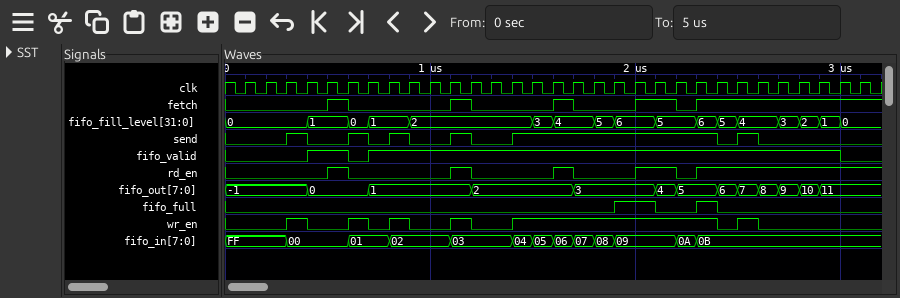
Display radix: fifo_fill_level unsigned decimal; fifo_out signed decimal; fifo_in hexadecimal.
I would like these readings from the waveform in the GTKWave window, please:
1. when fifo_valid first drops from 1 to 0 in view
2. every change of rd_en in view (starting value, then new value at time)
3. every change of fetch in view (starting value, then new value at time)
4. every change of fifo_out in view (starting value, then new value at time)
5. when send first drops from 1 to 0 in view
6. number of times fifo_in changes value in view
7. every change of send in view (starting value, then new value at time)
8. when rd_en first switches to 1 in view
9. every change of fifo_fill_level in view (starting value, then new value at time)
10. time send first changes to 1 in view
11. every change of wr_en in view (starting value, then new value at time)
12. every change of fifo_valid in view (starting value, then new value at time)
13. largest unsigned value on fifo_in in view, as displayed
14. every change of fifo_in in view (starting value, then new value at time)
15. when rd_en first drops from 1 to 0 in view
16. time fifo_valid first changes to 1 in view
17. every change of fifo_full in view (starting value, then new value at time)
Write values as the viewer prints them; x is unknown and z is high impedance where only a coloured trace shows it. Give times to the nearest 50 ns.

600 ns
0, 1 at 500 ns, 0 at 600 ns, 1 at 1100 ns, 0 at 1200 ns, 1 at 1600 ns, 0 at 1700 ns, 1 at 2000 ns, 0 at 2200 ns, 1 at 2300 ns
0, 1 at 500 ns, 0 at 600 ns, 1 at 1100 ns, 0 at 1200 ns, 1 at 1600 ns, 0 at 1700 ns, 1 at 2000 ns, 0 at 2200 ns, 1 at 2300 ns
-1, 0 at 400 ns, 1 at 700 ns, 2 at 1200 ns, 3 at 1700 ns, 4 at 2100 ns, 5 at 2200 ns, 6 at 2400 ns, 7 at 2500 ns, 8 at 2600 ns, 9 at 2700 ns, 10 at 2800 ns, 11 at 2900 ns
400 ns
12
0, 1 at 300 ns, 0 at 400 ns, 1 at 600 ns, 0 at 700 ns, 1 at 800 ns, 0 at 900 ns, 1 at 1100 ns, 0 at 1200 ns, 1 at 1400 ns, 0 at 2400 ns, 1 at 2500 ns, 0 at 2600 ns
500 ns
0, 1 at 400 ns, 0 at 600 ns, 1 at 700 ns, 2 at 900 ns, 3 at 1500 ns, 4 at 1600 ns, 5 at 1800 ns, 6 at 1900 ns, 5 at 2100 ns, 6 at 2300 ns, 5 at 2400 ns, 4 at 2500 ns, 3 at 2700 ns, 2 at 2800 ns, 1 at 2900 ns, 0 at 3000 ns
300 ns
0, 1 at 300 ns, 0 at 400 ns, 1 at 600 ns, 0 at 700 ns, 1 at 800 ns, 0 at 900 ns, 1 at 1100 ns, 0 at 1200 ns, 1 at 1400 ns, 0 at 2400 ns, 1 at 2500 ns, 0 at 2600 ns
0, 1 at 400 ns, 0 at 600 ns, 1 at 700 ns, 0 at 3000 ns
FF
FF, 00 at 300 ns, 01 at 600 ns, 02 at 800 ns, 03 at 1100 ns, 04 at 1400 ns, 05 at 1500 ns, 06 at 1600 ns, 07 at 1700 ns, 08 at 1800 ns, 09 at 1900 ns, 0A at 2200 ns, 0B at 2300 ns
600 ns
400 ns
0, 1 at 1900 ns, 0 at 2100 ns, 1 at 2300 ns, 0 at 2400 ns
